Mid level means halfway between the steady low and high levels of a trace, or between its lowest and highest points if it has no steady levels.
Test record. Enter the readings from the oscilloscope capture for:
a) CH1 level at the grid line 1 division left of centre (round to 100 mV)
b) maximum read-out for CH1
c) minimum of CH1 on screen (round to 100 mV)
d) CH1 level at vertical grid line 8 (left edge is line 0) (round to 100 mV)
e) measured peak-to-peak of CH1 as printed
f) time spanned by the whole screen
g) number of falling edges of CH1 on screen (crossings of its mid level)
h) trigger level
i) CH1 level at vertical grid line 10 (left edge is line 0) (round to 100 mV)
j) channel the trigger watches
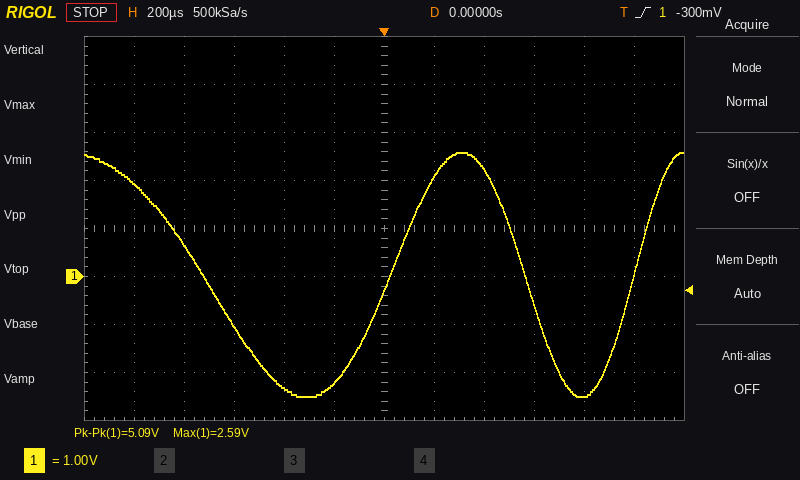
-2.2 V
2.59 V
-2.5 V
2.2 V
5.09 V
2.4 ms
2
-300 mV
-2.5 V
CH1
